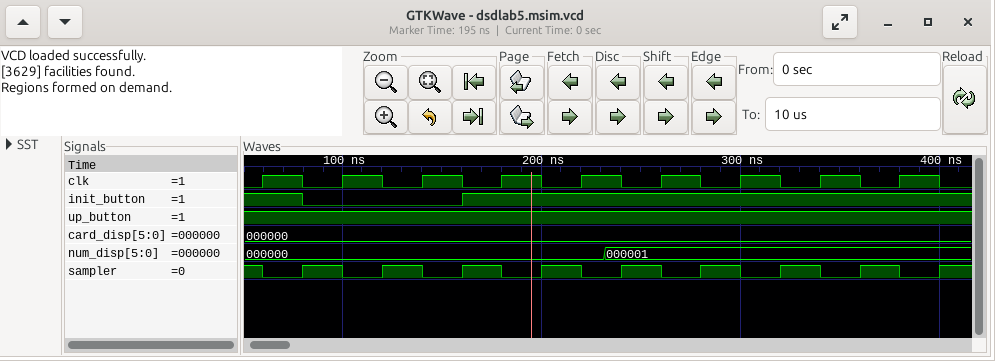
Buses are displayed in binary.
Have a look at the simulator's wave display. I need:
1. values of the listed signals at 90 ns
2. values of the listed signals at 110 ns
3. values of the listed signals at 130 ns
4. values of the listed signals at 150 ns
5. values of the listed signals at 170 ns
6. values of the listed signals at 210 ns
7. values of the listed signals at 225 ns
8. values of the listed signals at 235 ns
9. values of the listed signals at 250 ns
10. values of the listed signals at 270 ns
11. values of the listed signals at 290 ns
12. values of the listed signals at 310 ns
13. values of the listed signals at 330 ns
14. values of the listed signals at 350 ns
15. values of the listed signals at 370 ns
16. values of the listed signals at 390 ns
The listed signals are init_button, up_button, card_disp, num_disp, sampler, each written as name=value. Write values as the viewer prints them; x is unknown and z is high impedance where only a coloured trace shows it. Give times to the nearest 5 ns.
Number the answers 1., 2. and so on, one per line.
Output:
1. init_button=0, up_button=1, card_disp=000000, num_disp=000000, sampler=1
2. init_button=0, up_button=1, card_disp=000000, num_disp=000000, sampler=0
3. init_button=0, up_button=1, card_disp=000000, num_disp=000000, sampler=1
4. init_button=0, up_button=1, card_disp=000000, num_disp=000000, sampler=0
5. init_button=1, up_button=1, card_disp=000000, num_disp=000000, sampler=1
6. init_button=1, up_button=1, card_disp=000000, num_disp=000000, sampler=1
7. init_button=1, up_button=1, card_disp=000000, num_disp=000000, sampler=0
8. init_button=1, up_button=1, card_disp=000000, num_disp=000001, sampler=0
9. init_button=1, up_button=1, card_disp=000000, num_disp=000001, sampler=1
10. init_button=1, up_button=1, card_disp=000000, num_disp=000001, sampler=0
11. init_button=1, up_button=1, card_disp=000000, num_disp=000001, sampler=1
12. init_button=1, up_button=1, card_disp=000000, num_disp=000001, sampler=0
13. init_button=1, up_button=1, card_disp=000000, num_disp=000001, sampler=1
14. init_button=1, up_button=1, card_disp=000000, num_disp=000001, sampler=0
15. init_button=1, up_button=1, card_disp=000000, num_disp=000001, sampler=1
16. init_button=1, up_button=1, card_disp=000000, num_disp=000001, sampler=0
